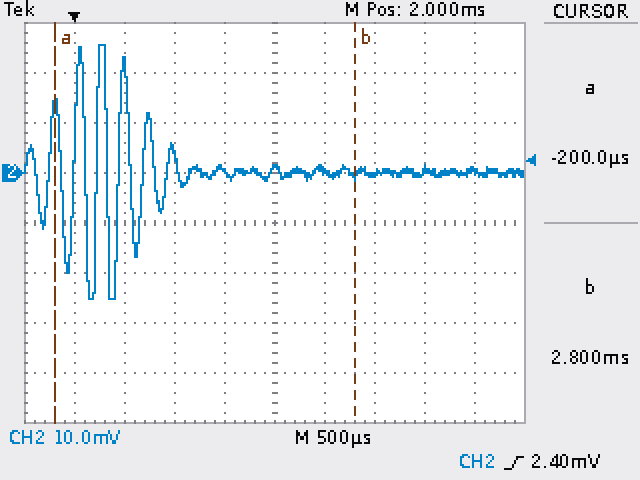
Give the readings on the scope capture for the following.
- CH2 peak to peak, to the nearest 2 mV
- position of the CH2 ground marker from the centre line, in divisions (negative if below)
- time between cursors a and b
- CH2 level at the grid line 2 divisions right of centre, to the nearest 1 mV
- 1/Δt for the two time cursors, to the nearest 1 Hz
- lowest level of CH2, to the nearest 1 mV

50 mV
+1.0 div
3.00 ms
0 mV
333 Hz
-25 mV
